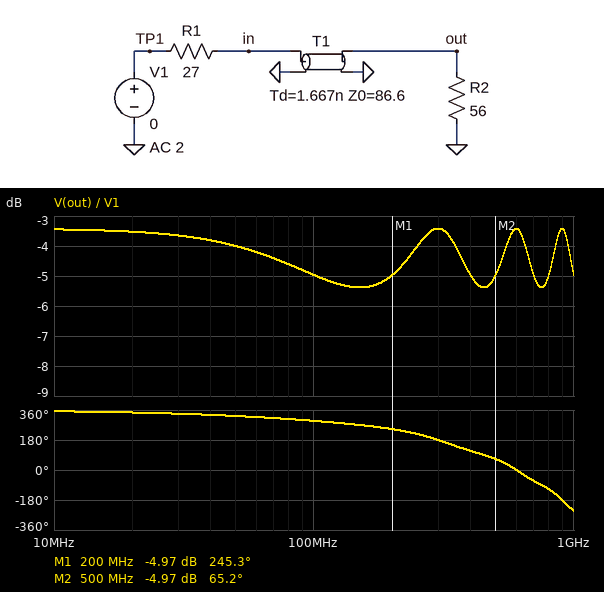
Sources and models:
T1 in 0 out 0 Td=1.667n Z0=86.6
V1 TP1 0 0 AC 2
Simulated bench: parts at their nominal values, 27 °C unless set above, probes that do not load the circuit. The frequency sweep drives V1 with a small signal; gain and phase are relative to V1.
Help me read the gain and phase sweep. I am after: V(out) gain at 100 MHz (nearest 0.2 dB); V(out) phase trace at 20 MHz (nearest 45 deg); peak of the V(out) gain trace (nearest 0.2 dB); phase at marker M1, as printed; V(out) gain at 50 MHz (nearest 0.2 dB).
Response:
-5.0 dB
360 deg
-3.4 dB
245.3 deg
-4.0 dB
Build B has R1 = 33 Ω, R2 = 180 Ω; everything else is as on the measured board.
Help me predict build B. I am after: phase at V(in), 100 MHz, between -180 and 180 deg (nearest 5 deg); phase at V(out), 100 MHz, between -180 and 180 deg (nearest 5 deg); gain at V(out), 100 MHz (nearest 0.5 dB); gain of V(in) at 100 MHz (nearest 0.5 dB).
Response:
-10 deg
-50 deg
0.5 dB
-3.5 dB
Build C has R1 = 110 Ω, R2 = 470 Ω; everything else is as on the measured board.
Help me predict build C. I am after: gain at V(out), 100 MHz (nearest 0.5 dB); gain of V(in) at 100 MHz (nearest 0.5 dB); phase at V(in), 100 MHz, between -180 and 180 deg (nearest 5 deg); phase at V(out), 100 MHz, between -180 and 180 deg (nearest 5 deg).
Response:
-3.0 dB
-8.5 dB
-45 deg
-65 deg
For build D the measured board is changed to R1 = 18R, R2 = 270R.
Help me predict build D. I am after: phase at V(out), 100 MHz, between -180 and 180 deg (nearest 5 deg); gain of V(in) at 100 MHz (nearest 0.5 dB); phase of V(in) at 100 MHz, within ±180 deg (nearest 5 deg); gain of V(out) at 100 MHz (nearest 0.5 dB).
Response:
-40 deg
-2.0 dB
-10 deg
3.0 dB
